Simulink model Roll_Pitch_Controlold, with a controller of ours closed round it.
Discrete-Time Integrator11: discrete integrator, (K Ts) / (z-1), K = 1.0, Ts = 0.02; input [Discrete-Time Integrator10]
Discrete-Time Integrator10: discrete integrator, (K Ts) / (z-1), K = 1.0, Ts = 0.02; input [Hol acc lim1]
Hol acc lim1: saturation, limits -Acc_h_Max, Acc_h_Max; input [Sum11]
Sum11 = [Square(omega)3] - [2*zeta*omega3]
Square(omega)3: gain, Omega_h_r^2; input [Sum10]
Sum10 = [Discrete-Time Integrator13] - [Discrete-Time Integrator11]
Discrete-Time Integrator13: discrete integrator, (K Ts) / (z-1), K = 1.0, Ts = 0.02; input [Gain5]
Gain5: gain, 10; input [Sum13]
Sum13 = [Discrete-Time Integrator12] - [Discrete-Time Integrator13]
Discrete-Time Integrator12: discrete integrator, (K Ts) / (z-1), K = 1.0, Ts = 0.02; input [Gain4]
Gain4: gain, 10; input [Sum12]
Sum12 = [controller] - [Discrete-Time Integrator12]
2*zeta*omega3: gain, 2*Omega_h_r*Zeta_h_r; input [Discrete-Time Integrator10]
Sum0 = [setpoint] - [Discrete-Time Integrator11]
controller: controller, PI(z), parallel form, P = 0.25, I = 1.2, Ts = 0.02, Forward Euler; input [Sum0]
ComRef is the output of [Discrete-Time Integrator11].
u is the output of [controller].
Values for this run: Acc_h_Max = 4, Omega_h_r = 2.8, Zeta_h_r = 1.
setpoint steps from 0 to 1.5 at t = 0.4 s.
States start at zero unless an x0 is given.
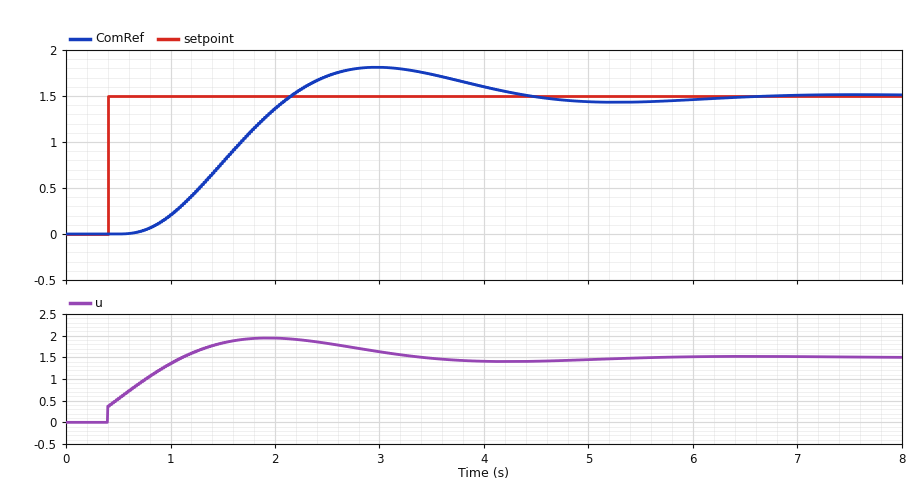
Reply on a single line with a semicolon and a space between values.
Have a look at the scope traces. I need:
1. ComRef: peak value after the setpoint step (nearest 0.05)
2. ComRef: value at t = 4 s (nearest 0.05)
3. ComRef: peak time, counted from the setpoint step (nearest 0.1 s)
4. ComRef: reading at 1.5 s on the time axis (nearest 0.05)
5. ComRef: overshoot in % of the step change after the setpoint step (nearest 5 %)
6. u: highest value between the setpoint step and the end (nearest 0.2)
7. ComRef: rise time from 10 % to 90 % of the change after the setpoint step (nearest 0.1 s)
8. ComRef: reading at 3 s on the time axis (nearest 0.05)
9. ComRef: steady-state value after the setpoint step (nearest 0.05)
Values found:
1.80; 1.60; 2.6 s; 0.80; 20 %; 2.0; 1.1 s; 1.80; 1.50
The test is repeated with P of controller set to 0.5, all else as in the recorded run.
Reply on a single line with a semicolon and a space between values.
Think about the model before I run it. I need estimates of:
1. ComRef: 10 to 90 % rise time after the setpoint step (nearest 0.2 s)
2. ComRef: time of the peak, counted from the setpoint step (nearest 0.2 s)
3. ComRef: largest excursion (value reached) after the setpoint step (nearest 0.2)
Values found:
1.0 s; 2.2 s; 1.6
